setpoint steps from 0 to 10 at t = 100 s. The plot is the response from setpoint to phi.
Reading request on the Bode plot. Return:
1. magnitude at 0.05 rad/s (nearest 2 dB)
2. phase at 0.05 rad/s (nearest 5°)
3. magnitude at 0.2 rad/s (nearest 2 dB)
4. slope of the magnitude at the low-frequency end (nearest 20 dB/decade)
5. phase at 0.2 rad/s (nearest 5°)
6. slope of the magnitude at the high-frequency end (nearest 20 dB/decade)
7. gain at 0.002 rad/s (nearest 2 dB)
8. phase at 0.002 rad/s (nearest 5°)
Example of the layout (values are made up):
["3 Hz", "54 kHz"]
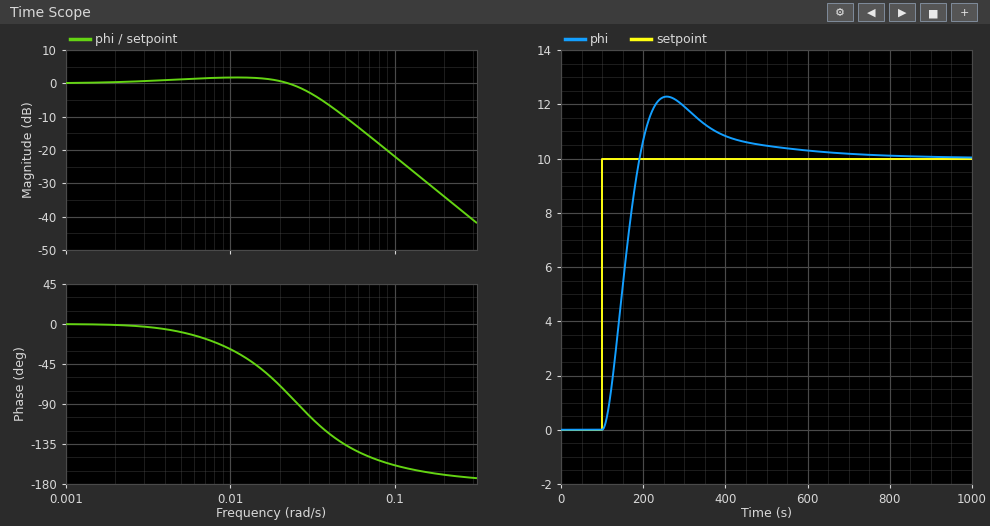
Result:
["-10 dB", "-135°", "-34 dB", "0 dB/decade", "-170°", "-40 dB/decade", "0 dB", "0°"]
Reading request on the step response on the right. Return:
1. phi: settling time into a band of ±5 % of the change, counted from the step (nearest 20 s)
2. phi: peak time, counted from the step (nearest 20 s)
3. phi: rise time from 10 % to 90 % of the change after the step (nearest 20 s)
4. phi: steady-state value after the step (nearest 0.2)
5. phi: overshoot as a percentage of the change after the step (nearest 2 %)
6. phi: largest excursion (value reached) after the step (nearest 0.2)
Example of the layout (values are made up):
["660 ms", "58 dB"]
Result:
["380 s", "160 s", "60 s", "10.0", "22 %", "12.2"]
